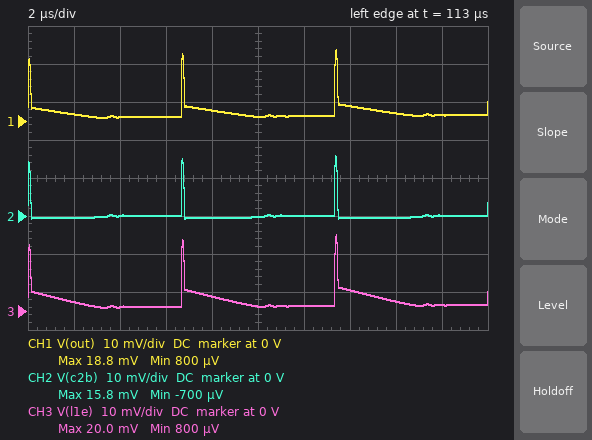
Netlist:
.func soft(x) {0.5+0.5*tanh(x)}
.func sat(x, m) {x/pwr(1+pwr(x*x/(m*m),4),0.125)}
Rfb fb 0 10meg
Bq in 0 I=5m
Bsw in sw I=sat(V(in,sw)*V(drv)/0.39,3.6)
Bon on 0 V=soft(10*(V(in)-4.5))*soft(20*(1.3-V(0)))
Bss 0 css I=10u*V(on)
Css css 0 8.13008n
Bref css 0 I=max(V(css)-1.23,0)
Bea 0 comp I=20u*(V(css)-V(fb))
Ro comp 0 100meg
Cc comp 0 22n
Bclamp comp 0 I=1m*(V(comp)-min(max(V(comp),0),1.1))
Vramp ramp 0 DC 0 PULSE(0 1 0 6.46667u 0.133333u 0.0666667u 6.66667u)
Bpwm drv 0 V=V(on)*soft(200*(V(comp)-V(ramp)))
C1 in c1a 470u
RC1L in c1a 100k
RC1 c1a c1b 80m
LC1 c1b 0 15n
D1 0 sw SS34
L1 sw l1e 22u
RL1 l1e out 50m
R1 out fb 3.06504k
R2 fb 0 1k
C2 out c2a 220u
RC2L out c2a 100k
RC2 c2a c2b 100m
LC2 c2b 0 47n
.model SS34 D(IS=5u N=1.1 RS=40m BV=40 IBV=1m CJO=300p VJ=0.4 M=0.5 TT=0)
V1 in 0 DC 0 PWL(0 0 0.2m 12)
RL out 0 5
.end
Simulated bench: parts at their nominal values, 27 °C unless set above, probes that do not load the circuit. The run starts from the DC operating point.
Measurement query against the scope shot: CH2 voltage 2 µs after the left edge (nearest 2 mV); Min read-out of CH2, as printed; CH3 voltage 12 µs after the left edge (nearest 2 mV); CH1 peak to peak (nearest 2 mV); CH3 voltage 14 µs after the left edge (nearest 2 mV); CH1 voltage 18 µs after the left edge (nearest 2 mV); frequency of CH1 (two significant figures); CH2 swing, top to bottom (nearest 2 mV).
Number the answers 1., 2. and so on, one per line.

1. 0 V
2. -700 µV
3. 2 mV
4. 18 mV
5. 6 mV
6. 2 mV
7. 150 kHz
8. 16 mV
